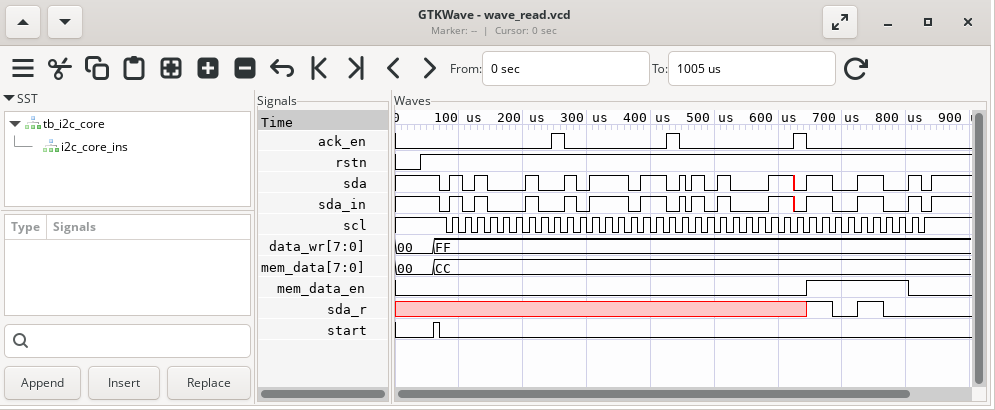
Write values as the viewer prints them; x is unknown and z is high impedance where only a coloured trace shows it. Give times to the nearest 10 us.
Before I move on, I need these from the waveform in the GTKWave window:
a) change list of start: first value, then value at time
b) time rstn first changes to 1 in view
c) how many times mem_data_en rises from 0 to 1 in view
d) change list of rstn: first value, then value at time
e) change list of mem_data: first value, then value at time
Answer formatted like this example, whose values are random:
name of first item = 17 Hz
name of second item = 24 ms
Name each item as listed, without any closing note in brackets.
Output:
change list of start: first value, then value at time = 0, 1 at 60 us, 0 at 70 us
time rstn first changes to 1 in view = 40 us
how many times mem_data_en rises from 0 to 1 in view = 1
change list of rstn: first value, then value at time = 0, 1 at 40 us
change list of mem_data: first value, then value at time = 00, CC at 60 us
